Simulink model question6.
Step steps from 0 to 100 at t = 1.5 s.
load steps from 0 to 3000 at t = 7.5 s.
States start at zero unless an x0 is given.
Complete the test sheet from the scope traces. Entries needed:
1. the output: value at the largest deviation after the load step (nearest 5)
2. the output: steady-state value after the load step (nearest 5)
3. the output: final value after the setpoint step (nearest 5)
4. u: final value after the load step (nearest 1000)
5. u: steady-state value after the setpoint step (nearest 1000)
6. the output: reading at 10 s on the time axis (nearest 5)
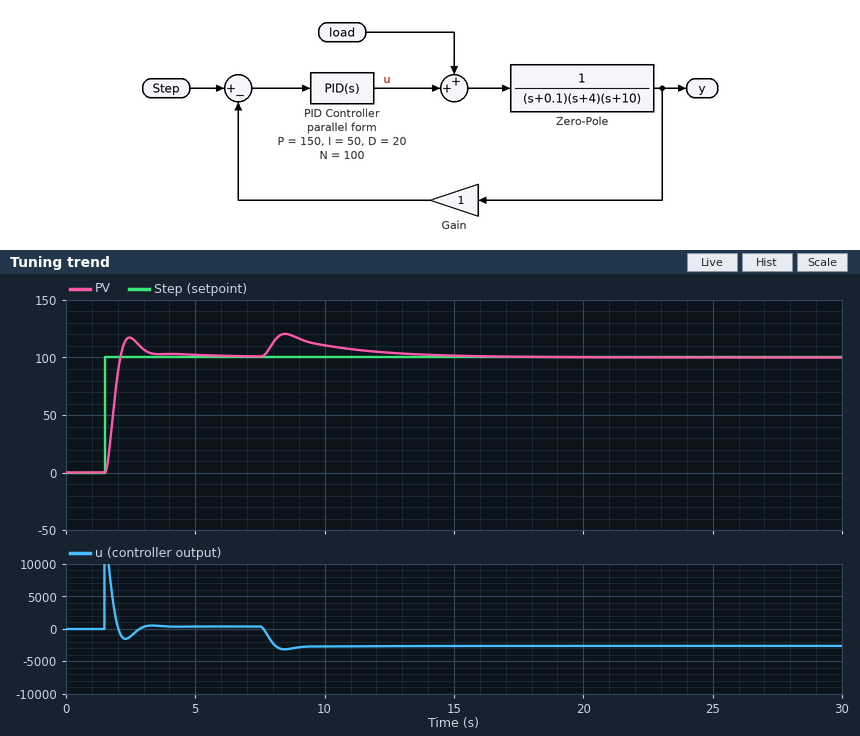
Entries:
120
100
100
-3000
0
110
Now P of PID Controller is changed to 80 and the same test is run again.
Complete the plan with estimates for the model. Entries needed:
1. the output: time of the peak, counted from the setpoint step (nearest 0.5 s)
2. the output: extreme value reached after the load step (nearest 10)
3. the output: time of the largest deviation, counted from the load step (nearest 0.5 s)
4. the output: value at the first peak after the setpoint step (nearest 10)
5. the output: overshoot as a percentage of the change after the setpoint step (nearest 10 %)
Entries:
2.0 s
130
1.5 s
120
20 %
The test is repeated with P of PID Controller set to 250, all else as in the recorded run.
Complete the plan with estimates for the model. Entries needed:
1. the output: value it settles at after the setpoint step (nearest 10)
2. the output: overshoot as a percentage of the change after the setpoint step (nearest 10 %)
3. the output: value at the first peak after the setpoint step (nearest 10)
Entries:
100
30 %
130
